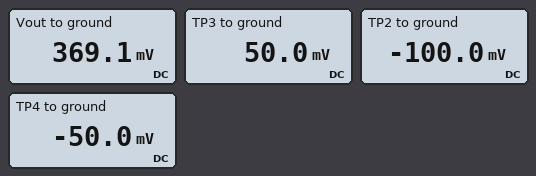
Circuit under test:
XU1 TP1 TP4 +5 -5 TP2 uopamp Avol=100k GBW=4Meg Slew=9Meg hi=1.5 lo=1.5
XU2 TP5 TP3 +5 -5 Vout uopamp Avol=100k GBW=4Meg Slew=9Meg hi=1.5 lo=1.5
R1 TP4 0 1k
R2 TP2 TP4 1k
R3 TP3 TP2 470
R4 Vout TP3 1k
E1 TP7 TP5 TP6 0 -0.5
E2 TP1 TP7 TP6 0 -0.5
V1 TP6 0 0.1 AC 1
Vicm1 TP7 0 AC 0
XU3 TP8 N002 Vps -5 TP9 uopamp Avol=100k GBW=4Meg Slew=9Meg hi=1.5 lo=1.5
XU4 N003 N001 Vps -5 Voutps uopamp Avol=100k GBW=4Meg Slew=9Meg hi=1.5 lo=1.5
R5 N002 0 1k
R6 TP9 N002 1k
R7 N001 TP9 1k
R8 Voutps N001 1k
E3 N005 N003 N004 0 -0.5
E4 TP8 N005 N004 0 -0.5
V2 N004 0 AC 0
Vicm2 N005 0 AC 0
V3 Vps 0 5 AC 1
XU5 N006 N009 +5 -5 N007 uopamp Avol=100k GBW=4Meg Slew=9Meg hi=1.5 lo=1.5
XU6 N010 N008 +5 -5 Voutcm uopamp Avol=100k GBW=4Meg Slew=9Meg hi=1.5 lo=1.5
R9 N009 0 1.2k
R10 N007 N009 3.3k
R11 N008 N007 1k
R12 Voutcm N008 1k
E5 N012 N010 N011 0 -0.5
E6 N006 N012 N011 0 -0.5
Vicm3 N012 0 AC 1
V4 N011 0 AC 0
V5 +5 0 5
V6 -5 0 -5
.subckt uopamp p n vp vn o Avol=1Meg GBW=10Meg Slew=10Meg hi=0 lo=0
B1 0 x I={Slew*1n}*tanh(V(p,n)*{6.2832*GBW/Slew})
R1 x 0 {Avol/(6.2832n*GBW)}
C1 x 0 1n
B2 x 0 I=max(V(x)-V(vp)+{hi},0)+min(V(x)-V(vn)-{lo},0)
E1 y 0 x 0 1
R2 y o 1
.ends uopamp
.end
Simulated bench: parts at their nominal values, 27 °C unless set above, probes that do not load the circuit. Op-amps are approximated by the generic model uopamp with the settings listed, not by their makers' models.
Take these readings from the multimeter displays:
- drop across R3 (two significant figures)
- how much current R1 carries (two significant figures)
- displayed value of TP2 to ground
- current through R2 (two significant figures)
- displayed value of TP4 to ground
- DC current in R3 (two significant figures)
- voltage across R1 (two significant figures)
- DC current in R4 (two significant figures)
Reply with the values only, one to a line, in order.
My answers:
150 mV
50 µA
-100.0 mV
50 µA
-50.0 mV
320 µA
50 mV
320 µA
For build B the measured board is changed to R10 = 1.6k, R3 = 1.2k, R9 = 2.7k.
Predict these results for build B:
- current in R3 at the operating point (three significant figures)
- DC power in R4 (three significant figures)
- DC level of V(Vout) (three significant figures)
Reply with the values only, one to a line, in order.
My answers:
125 µA
15.6 µW
175 mV
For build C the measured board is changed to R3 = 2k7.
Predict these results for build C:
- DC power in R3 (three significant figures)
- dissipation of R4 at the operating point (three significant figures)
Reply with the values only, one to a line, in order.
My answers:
8.33 µW
3.09 µW
